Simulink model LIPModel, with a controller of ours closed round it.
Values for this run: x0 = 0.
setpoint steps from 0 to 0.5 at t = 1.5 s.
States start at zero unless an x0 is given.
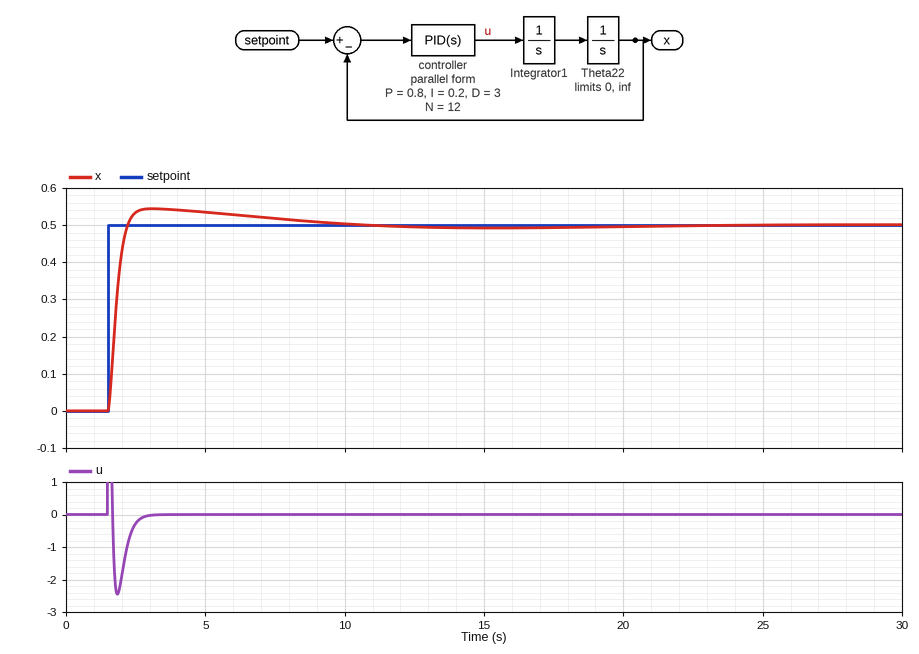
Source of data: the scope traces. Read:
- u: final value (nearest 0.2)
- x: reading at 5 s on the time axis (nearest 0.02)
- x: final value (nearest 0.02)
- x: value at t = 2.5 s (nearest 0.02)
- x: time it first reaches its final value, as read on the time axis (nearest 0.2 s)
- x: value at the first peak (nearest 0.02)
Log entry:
0.0
0.54
0.50
0.54
2.2 s
0.54
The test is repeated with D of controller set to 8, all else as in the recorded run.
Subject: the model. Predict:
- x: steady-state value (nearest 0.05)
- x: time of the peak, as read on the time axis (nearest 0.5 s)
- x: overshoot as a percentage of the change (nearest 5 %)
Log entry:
0.50
2.0 s
10 %
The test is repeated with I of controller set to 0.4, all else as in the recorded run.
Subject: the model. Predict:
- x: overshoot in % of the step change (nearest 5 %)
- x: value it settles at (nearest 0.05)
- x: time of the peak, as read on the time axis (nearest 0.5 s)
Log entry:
10 %
0.50
3.5 s
